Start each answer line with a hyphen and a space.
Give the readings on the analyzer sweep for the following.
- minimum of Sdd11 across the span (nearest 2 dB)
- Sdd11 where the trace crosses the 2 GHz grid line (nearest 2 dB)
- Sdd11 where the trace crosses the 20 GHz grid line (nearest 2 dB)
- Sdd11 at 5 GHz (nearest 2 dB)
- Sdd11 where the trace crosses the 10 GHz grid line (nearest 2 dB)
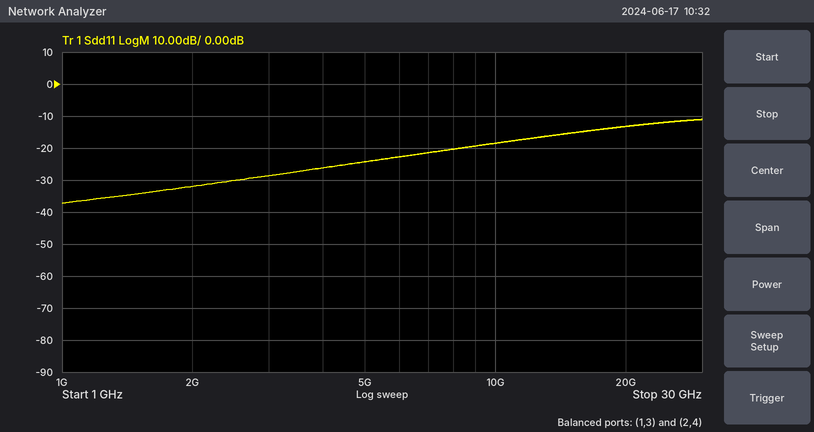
- -38 dB
- -32 dB
- -14 dB
- -24 dB
- -18 dB
